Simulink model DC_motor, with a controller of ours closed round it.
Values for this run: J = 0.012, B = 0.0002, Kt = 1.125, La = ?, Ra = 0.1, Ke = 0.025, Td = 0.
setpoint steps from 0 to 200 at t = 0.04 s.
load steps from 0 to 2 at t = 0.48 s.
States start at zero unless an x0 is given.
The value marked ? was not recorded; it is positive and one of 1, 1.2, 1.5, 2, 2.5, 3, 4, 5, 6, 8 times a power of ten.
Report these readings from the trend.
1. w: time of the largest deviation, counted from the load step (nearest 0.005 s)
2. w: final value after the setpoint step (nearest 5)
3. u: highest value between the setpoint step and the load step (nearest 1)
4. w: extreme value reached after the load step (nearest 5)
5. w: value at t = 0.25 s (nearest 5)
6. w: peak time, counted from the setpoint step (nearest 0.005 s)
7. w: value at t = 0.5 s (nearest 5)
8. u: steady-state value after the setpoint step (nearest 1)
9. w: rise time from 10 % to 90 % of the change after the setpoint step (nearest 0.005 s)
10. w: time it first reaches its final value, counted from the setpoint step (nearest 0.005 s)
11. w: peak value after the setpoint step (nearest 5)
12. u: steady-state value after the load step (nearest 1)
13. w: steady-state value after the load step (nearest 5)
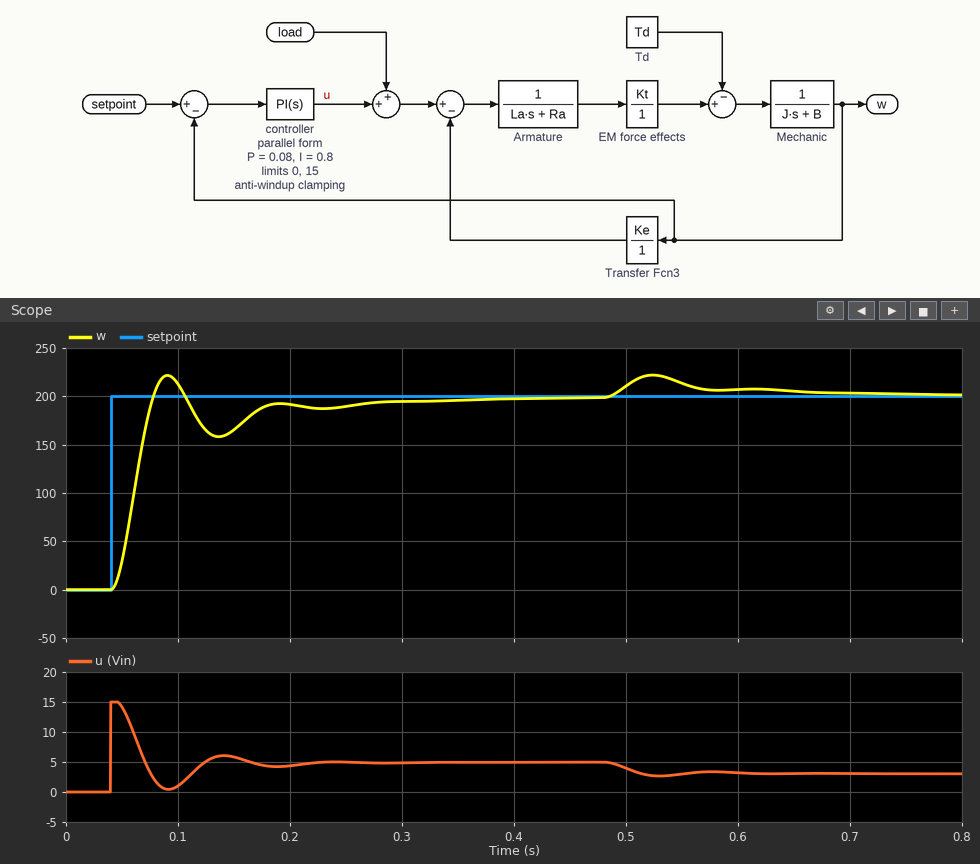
0.045 s
200
15
220
190
0.050 s
210
5
0.025 s
0.040 s
220
3
200
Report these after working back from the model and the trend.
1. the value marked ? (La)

0.002
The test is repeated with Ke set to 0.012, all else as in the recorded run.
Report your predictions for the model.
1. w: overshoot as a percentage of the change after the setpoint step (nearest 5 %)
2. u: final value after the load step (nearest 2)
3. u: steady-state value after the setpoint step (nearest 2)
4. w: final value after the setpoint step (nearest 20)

25 %
0
2
200
